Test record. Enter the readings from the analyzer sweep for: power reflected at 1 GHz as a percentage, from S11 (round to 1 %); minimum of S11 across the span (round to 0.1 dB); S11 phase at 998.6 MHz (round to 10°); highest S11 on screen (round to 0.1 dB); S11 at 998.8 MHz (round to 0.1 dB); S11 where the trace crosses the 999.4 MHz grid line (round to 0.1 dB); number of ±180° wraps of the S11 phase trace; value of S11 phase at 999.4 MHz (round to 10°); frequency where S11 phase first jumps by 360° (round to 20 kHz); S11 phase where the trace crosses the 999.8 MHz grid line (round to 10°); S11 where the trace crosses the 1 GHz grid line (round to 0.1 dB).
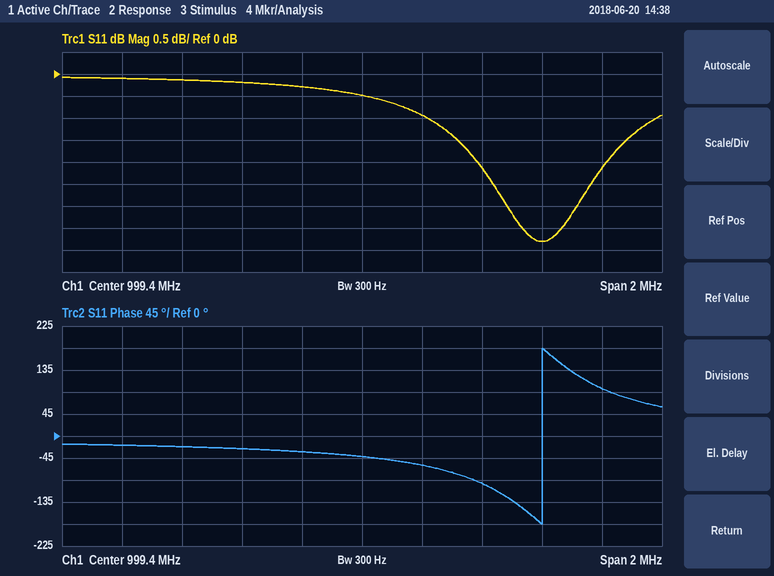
42 %
-3.8 dB
-20°
-0.1 dB
-0.1 dB
-0.5 dB
1
-40°
1.00000 GHz
-100°
-3.8 dB
